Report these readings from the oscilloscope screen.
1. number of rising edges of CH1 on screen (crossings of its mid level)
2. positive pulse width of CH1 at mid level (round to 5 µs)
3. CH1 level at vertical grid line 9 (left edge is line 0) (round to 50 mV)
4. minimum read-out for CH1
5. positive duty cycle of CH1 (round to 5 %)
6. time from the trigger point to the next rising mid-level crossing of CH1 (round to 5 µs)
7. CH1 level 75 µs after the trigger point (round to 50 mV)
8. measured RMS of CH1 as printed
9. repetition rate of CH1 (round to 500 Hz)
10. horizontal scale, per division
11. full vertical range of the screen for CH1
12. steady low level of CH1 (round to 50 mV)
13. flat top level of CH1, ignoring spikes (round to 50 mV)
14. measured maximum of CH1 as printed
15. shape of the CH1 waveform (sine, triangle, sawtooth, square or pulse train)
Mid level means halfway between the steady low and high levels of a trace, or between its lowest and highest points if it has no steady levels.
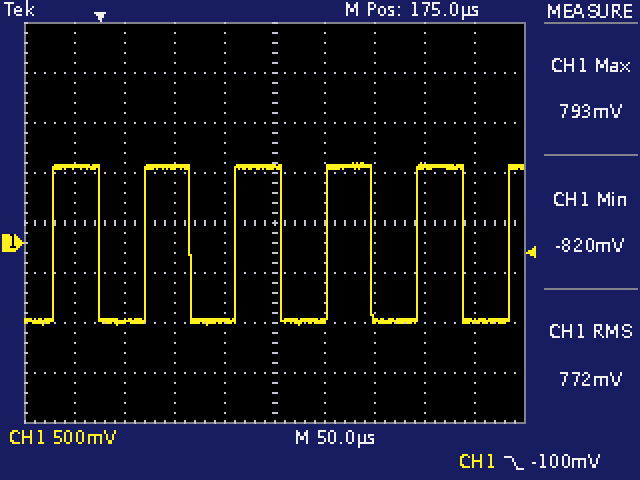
6
45 µs
-800 mV
-820 mV
50 %
45 µs
750 mV
772 mV
11.0 kHz
50 µs
4 V
-800 mV
750 mV
793 mV
square
